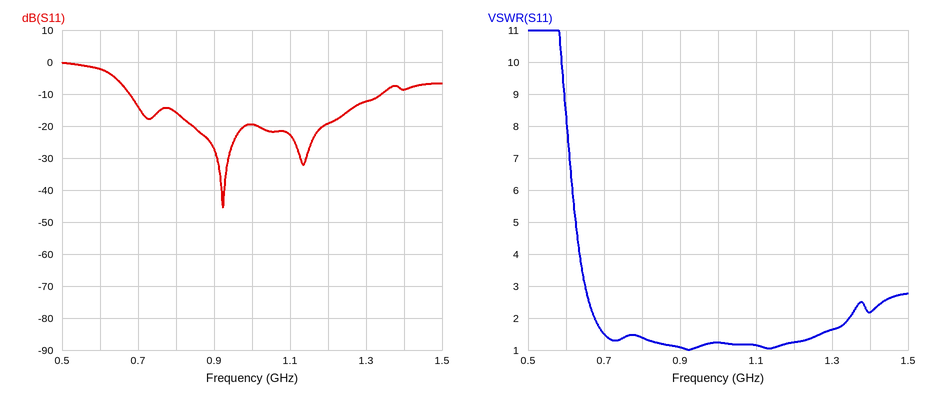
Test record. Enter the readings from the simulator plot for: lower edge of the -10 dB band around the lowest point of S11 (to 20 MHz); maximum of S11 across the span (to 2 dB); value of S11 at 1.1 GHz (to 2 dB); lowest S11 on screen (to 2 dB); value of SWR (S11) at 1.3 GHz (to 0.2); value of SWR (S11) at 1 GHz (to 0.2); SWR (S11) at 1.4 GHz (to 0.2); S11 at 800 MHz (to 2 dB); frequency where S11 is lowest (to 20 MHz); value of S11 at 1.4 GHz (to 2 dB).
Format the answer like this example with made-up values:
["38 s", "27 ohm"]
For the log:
["680 MHz", "0 dB", "-22 dB", "-46 dB", "1.6", "1.2", "2.2", "-16 dB", "920 MHz", "-8 dB"]
